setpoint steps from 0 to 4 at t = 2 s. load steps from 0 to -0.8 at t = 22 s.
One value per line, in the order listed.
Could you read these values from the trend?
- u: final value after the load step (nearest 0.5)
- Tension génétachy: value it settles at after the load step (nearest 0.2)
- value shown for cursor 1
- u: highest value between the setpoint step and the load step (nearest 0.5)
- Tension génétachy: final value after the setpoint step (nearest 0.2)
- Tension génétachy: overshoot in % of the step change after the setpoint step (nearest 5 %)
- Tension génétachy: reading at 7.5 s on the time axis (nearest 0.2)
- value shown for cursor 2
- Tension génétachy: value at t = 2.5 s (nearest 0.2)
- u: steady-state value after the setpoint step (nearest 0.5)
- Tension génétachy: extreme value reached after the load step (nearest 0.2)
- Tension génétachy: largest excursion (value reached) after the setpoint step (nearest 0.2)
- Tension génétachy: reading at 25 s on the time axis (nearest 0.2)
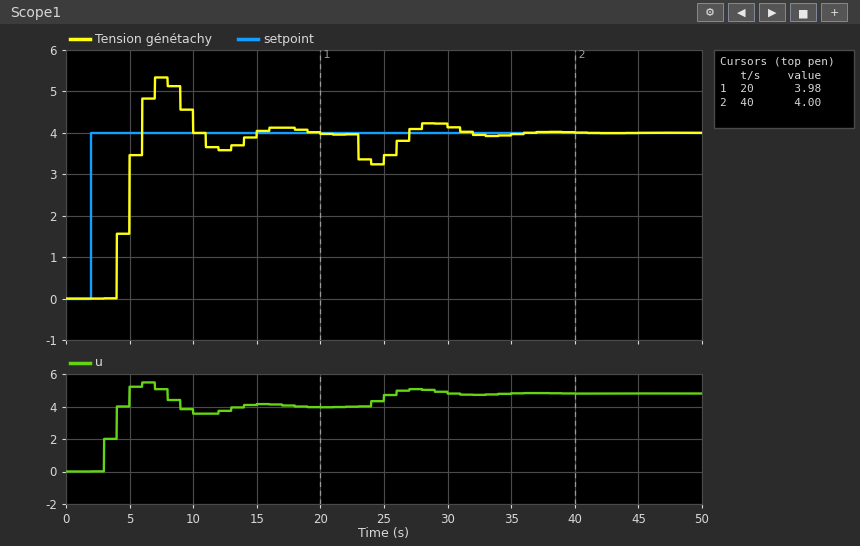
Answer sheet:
5.0
4.0
3.98
5.5
4.0
35 %
5.4
4.00
0.0
4.0
3.2
5.4
3.4
